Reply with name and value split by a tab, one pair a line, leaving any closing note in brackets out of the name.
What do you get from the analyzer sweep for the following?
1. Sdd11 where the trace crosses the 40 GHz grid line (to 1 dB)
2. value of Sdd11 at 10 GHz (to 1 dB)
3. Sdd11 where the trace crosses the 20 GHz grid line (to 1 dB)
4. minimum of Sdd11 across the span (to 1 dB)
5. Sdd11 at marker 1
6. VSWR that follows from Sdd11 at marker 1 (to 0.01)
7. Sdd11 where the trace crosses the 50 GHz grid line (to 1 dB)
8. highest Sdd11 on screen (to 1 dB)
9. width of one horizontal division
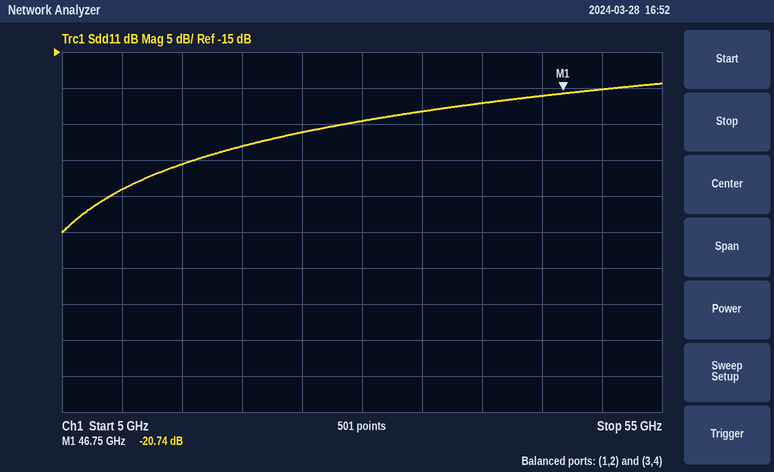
Sdd11 where the trace crosses the 40 GHz grid line	-22 dB
value of Sdd11 at 10 GHz	-34 dB
Sdd11 where the trace crosses the 20 GHz grid line	-28 dB
minimum of Sdd11 across the span	-40 dB
Sdd11 at marker 1	-20.74 dB
VSWR that follows from Sdd11 at marker 1	1.20
Sdd11 where the trace crosses the 50 GHz grid line	-20 dB
highest Sdd11 on screen	-19 dB
width of one horizontal division	5 GHz
